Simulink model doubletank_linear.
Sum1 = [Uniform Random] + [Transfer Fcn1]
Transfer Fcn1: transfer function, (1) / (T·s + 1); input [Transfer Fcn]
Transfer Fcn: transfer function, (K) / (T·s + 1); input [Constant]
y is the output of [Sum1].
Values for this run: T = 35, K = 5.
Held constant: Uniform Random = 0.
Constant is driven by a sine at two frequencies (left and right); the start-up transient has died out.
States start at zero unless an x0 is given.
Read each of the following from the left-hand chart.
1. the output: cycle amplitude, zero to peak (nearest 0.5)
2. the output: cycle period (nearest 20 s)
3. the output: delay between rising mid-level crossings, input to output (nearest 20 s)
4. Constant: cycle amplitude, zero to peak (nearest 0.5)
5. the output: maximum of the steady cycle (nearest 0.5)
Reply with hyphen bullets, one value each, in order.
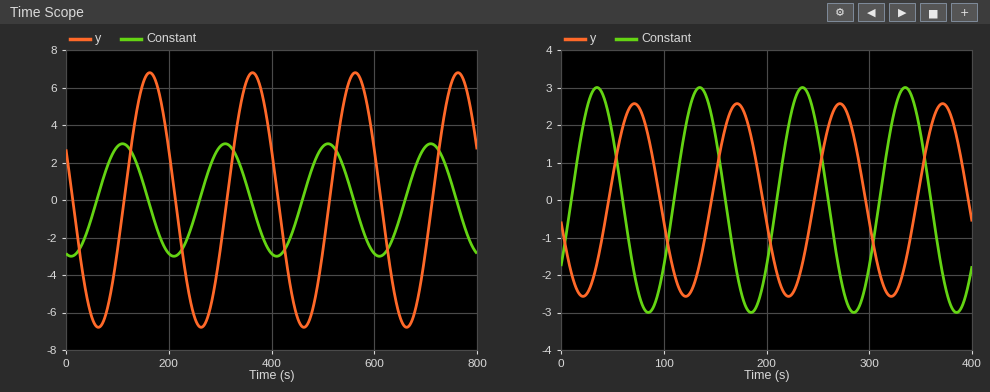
- 7.0
- 200 s
- 60 s
- 3.0
- 7.0
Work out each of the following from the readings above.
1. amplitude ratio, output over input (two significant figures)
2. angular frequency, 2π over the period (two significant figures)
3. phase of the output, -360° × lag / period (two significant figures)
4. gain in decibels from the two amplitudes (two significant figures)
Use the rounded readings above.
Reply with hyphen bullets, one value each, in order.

- 2.3
- 0.031 rad/s
- -110°
- 7.4 dB
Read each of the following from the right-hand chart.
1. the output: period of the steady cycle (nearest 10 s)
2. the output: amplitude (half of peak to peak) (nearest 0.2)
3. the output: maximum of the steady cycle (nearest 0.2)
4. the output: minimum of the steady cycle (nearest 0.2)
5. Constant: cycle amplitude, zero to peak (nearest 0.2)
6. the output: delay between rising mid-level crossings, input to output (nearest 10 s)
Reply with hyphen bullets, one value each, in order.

- 100 s
- 2.6
- 2.6
- -2.6
- 3.0
- 40 s
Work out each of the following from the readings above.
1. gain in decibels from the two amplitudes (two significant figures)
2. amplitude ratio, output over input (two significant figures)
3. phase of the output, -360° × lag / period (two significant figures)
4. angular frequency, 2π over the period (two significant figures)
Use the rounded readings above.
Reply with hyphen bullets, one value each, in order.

- -1.2 dB
- 0.87
- -140°
- 0.063 rad/s
